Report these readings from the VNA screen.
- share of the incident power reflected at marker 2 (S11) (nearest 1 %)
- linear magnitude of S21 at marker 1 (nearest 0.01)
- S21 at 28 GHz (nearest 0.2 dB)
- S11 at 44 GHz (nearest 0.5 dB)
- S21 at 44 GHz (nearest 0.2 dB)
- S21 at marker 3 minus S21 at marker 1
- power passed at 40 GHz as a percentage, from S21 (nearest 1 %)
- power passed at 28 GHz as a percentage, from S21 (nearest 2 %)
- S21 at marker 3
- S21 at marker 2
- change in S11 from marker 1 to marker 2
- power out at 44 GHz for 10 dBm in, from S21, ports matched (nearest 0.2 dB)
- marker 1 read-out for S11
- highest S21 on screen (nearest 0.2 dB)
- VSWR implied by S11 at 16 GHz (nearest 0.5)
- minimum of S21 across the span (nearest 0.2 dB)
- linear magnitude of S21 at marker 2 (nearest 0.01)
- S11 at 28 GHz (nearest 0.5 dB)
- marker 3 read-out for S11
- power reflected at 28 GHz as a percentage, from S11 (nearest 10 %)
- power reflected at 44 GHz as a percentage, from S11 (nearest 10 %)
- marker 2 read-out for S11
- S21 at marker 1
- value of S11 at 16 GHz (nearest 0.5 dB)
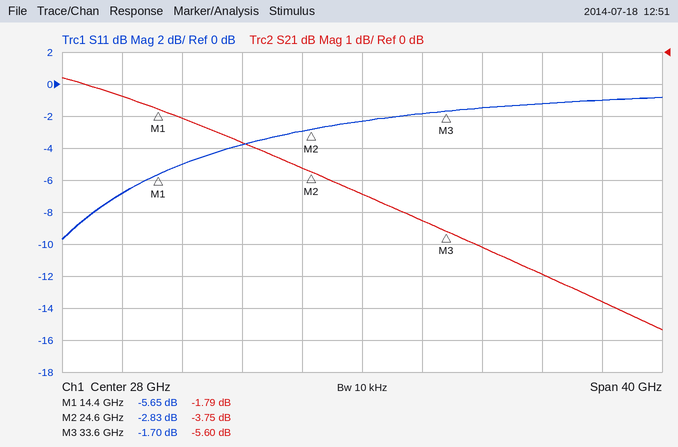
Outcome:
52 %
0.81
-4.4 dB
-1.0 dB
-7.8 dB
-3.81 dB
20 %
36 %
-5.60 dB
-3.75 dB
2.82 dB
2.2 dBm
-5.65 dB
-0.8 dB
3.5
-8.6 dB
0.65
-2.5 dB
-1.70 dB
60 %
80 %
-2.83 dB
-1.79 dB
-5.0 dB
